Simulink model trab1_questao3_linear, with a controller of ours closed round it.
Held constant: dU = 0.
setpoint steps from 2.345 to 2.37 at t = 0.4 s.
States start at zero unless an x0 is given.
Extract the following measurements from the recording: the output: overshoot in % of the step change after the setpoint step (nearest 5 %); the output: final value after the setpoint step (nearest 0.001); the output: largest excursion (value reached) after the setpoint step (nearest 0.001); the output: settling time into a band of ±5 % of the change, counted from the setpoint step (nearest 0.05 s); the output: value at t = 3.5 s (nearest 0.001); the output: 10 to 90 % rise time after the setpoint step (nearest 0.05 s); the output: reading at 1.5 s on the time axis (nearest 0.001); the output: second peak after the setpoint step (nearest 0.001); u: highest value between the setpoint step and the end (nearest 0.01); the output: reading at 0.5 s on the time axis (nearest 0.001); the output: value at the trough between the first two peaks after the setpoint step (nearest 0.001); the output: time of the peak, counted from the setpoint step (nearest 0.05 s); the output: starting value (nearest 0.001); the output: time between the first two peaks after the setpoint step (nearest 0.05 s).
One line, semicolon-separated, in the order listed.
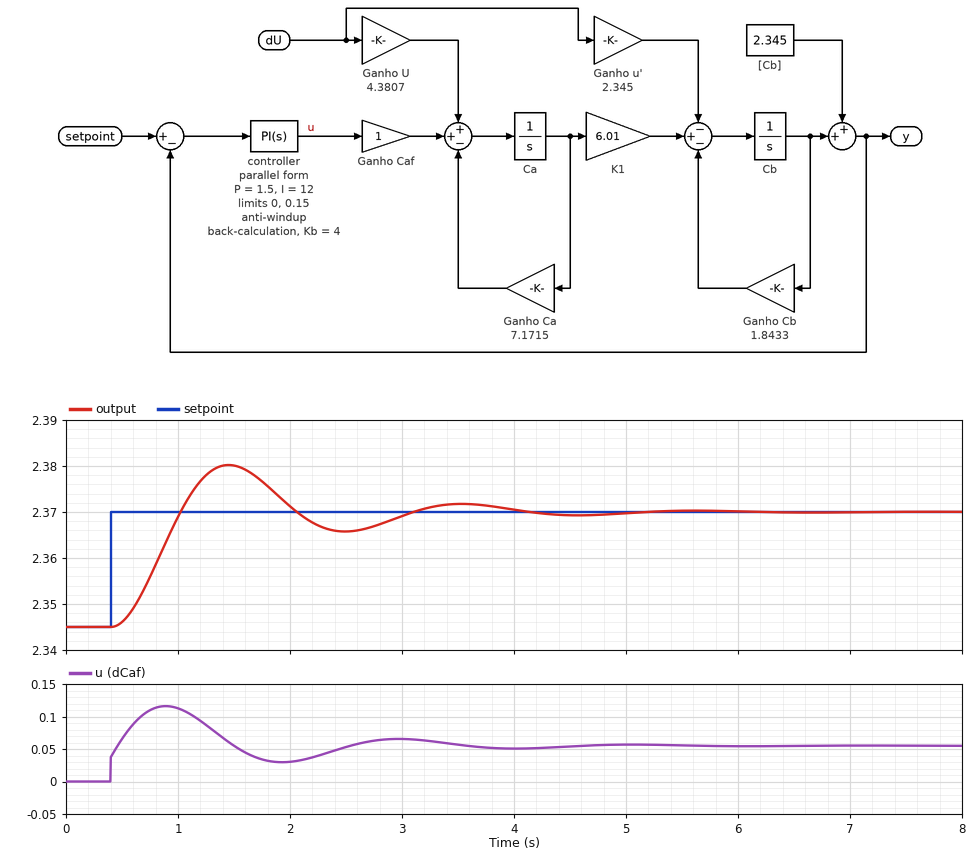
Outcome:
40 %; 2.370; 2.380; 3.40 s; 2.372; 0.40 s; 2.380; 2.372; 0.12; 2.346; 2.366; 1.05 s; 2.345; 2.10 s
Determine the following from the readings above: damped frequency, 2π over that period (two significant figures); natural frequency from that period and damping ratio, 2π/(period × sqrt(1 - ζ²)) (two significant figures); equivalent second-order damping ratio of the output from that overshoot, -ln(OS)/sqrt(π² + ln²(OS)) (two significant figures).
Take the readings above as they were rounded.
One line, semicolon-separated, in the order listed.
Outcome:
3.0 rad/s; 3.1 rad/s; 0.28
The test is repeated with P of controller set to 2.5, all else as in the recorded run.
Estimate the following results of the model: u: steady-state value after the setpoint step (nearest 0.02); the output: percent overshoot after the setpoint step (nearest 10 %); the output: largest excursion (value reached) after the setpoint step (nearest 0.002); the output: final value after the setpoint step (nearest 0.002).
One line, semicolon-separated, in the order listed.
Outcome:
0.06; 30 %; 2.378; 2.370
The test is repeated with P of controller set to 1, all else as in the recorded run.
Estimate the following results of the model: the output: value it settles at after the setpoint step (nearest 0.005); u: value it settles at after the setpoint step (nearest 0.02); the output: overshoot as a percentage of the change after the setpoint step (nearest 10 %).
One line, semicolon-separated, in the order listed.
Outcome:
2.370; 0.06; 50 %
